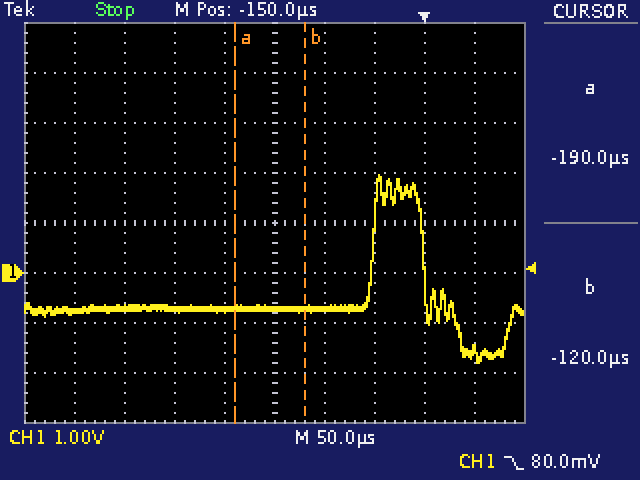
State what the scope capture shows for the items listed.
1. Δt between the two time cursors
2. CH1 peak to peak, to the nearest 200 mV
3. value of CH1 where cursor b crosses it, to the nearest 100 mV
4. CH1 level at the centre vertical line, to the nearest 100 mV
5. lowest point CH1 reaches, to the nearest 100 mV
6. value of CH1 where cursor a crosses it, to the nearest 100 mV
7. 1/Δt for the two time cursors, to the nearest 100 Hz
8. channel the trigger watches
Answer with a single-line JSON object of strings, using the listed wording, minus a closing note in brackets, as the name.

{"Δt between the two time cursors": "70 µs", "CH1 peak to peak, to the nearest 200 mV": "3.8 V", "value of CH1 where cursor b crosses it, to the nearest 100 mV": "-700 mV", "CH1 level at the centre vertical line, to the nearest 100 mV": "-700 mV", "lowest point CH1 reaches, to the nearest 100 mV": "-1.8 V", "value of CH1 where cursor a crosses it, to the nearest 100 mV": "-700 mV", "1/Δt for the two time cursors, to the nearest 100 Hz": "14.3 kHz", "channel the trigger watches": "CH1"}
